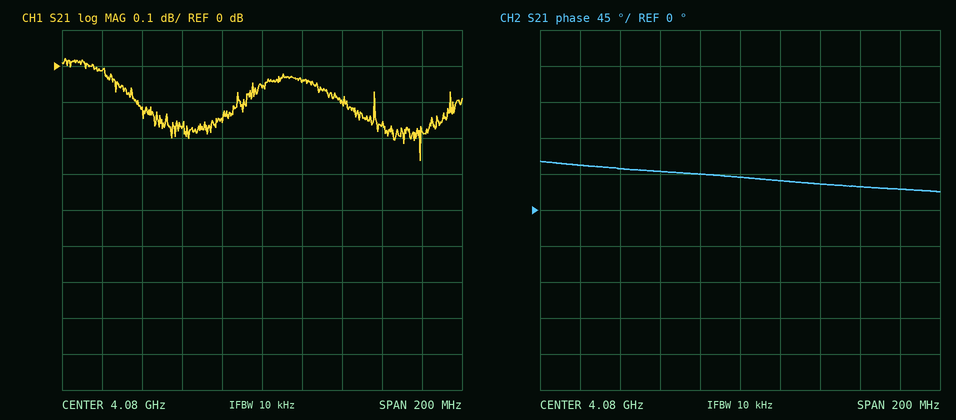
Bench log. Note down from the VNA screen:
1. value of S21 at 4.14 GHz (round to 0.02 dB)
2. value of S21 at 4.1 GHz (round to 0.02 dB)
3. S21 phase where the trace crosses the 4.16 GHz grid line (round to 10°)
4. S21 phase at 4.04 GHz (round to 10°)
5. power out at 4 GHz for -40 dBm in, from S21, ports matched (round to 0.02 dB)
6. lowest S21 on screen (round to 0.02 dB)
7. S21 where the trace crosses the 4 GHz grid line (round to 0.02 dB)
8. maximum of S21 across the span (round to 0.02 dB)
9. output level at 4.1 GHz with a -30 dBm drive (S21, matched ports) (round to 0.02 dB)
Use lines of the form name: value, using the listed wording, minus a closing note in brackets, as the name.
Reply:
value of S21 at 4.14 GHz: -0.16 dB
value of S21 at 4.1 GHz: -0.04 dB
S21 phase where the trace crosses the 4.16 GHz grid line: 30°
S21 phase at 4.04 GHz: 50°
power out at 4 GHz for -40 dBm in, from S21, ports matched: -40.02 dBm
lowest S21 on screen: -0.26 dB
S21 where the trace crosses the 4 GHz grid line: -0.02 dB
maximum of S21 across the span: 0.02 dB
output level at 4.1 GHz with a -30 dBm drive (S21, matched ports): -30.04 dBm
